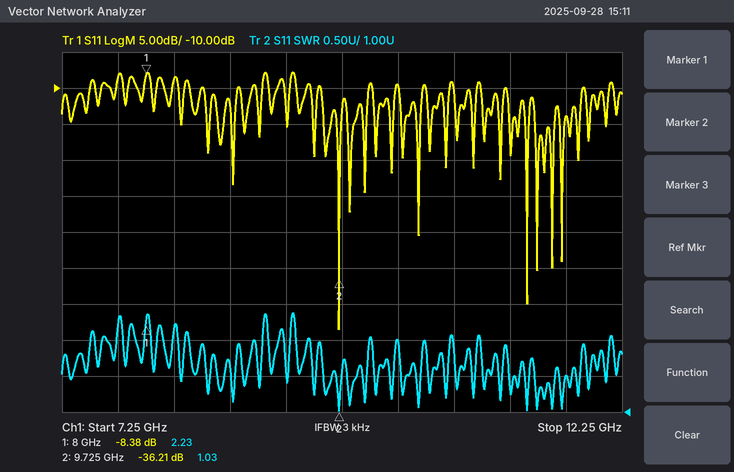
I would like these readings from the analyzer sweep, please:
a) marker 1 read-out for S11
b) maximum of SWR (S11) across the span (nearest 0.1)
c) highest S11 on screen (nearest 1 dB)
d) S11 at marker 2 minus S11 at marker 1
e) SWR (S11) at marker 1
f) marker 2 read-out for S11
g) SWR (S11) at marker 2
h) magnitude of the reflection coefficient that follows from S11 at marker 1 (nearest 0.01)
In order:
-8.38 dB
2.4
-8 dB
-27.83 dB
2.23
-36.21 dB
1.03
0.38
